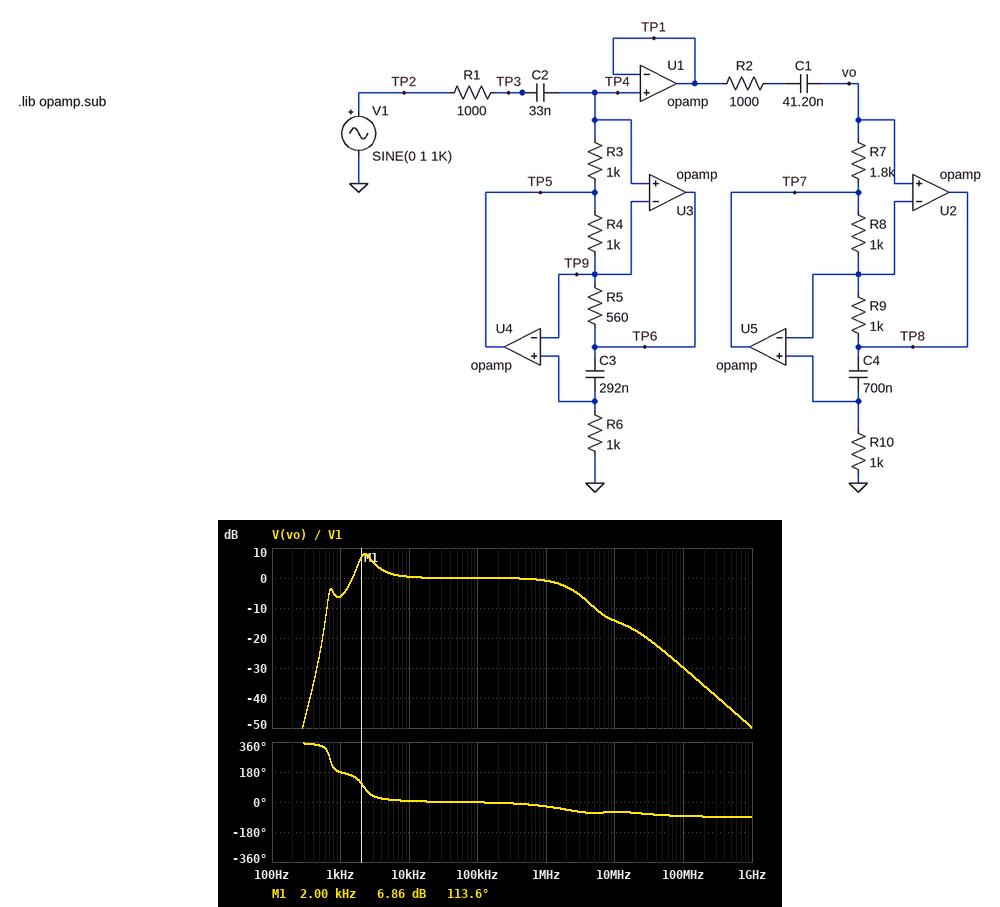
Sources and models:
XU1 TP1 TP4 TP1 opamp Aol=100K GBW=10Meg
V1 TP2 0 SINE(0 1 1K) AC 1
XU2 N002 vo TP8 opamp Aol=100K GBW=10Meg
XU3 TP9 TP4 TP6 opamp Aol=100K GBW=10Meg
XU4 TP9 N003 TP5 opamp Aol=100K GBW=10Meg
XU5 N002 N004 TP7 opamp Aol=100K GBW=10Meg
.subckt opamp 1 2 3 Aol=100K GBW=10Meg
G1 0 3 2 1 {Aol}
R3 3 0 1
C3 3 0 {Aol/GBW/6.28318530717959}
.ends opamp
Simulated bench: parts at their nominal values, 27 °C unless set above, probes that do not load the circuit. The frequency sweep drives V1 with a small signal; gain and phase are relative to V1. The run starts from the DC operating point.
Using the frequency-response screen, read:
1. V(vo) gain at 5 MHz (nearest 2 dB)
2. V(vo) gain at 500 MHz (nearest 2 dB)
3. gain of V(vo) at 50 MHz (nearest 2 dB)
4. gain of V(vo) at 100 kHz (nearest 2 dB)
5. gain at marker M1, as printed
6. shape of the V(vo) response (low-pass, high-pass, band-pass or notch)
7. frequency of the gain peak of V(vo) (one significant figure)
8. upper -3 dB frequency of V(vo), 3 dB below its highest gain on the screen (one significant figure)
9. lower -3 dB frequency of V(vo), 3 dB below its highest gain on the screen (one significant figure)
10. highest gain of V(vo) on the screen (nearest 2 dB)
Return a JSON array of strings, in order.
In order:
["-10 dB", "-44 dB", "-24 dB", "0 dB", "6.86 dB", "band-pass", "2 kHz", "3 kHz", "2 kHz", "8 dB"]
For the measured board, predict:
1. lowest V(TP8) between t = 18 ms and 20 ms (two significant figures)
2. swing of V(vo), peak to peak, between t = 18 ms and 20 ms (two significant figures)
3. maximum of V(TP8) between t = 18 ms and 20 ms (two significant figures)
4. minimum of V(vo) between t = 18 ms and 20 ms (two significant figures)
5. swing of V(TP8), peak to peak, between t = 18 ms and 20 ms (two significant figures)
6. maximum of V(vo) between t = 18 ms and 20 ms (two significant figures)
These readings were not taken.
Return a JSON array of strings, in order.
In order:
["-510 mV", "990 mV", "510 mV", "-500 mV", "1.0 V", "500 mV"]
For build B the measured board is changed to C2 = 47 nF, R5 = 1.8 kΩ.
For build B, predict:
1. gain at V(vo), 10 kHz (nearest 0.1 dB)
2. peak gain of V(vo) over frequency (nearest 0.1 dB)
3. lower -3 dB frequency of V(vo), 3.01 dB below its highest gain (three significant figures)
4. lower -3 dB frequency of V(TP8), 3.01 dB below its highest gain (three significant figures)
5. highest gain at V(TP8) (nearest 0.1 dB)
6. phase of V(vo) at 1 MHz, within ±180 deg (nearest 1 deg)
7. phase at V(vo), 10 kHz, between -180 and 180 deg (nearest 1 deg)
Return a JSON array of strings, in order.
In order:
["0.1 dB", "15.9 dB", "691 Hz", "688 Hz", "16.1 dB", "-21 deg", "2 deg"]
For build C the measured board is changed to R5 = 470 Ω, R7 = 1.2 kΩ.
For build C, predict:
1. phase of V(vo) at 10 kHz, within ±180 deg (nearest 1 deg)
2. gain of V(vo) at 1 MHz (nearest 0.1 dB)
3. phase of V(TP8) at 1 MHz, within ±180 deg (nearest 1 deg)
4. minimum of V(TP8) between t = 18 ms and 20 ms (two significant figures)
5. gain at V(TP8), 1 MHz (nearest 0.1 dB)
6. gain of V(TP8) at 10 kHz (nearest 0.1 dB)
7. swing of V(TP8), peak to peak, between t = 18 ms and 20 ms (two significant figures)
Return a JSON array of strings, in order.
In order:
["8 deg", "-1.2 dB", "-31 deg", "-660 mV", "-1.0 dB", "0.5 dB", "1.3 V"]
